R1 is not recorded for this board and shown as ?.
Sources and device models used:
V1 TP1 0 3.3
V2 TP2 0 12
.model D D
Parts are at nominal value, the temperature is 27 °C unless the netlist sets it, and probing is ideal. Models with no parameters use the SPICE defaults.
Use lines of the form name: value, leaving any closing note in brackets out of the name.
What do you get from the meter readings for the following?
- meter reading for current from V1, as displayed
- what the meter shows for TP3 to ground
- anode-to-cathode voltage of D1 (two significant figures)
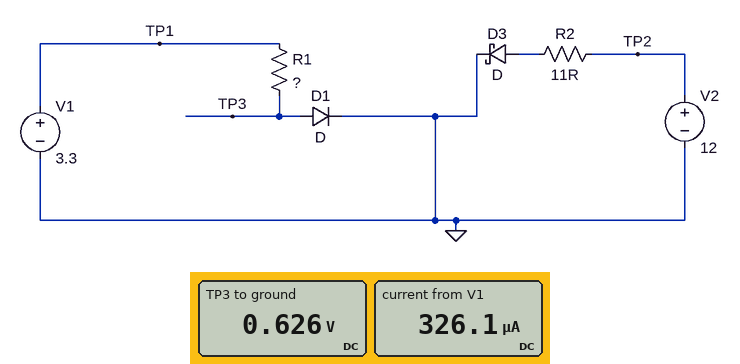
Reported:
meter reading for current from V1, as displayed: 326.1 µA
what the meter shows for TP3 to ground: 0.626 V
anode-to-cathode voltage of D1: 630 mV
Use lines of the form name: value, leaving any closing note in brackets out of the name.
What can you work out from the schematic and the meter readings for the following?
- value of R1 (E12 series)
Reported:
value of R1: 8.2 kΩ
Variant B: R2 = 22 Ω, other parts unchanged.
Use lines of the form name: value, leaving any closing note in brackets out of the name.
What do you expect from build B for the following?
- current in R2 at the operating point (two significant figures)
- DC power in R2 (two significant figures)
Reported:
current in R2 at the operating point: 510 mA
DC power in R2: 5.7 W
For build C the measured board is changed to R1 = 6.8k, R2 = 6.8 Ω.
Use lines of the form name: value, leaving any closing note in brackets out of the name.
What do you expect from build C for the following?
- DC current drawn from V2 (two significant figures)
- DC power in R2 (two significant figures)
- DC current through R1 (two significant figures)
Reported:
DC current drawn from V2: 1.6 A
DC power in R2: 18 W
DC current through R1: 390 µA
